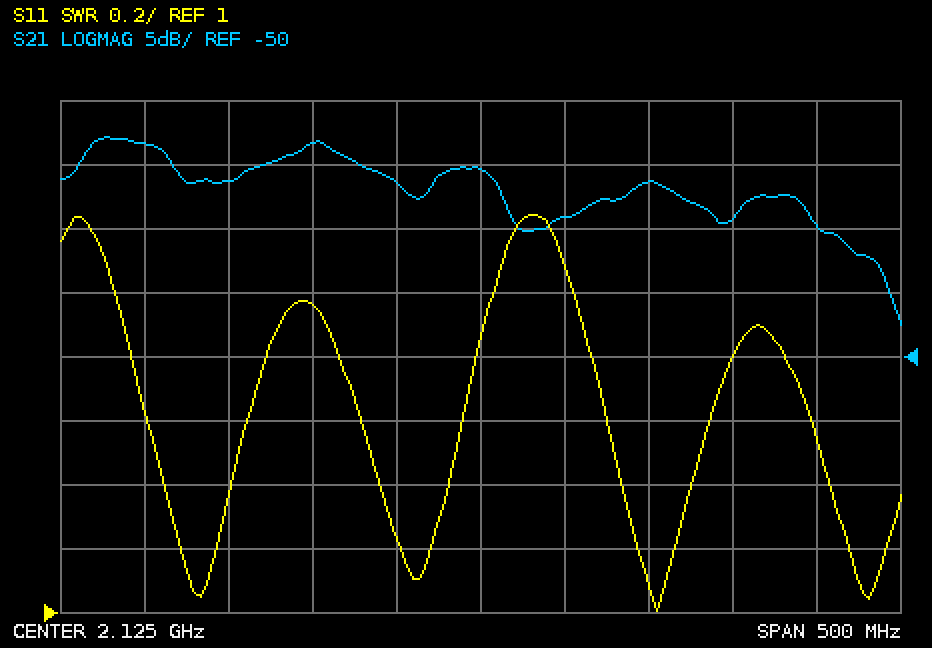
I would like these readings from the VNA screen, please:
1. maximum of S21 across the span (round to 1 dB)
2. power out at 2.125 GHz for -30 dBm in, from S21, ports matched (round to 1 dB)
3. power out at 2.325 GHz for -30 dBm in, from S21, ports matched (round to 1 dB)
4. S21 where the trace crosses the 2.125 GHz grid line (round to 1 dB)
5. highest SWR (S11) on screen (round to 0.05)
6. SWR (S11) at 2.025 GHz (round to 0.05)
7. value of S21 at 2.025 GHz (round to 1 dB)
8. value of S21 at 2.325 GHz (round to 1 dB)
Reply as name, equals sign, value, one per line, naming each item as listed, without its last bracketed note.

maximum of S21 across the span = -33 dB
power out at 2.125 GHz for -30 dBm in, from S21, ports matched = -65 dBm
power out at 2.325 GHz for -30 dBm in, from S21, ports matched = -70 dBm
S21 where the trace crosses the 2.125 GHz grid line = -35 dB
highest SWR (S11) on screen = 2.25
SWR (S11) at 2.025 GHz = 1.95
value of S21 at 2.025 GHz = -33 dB
value of S21 at 2.325 GHz = -40 dB
